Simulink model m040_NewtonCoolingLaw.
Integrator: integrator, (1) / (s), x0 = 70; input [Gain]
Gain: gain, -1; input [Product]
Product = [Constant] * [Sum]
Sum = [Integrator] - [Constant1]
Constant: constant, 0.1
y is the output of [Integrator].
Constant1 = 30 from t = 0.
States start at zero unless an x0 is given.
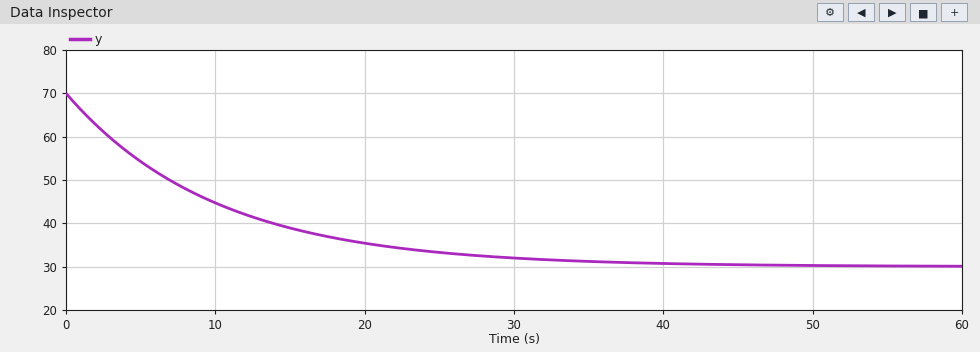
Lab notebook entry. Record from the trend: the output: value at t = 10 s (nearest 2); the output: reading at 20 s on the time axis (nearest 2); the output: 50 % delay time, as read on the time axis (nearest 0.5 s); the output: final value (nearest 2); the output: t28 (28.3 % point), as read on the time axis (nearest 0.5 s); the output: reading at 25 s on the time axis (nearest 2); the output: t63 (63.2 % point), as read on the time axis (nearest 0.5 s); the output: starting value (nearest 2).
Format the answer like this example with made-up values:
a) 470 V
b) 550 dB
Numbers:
a) 44
b) 36
c) 7.0 s
d) 30
e) 3.5 s
f) 34
g) 10.0 s
h) 70
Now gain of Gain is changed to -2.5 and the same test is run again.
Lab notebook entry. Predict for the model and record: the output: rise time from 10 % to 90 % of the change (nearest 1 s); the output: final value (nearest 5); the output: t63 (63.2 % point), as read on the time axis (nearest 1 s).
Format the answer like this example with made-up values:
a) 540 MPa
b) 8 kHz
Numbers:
a) 9 s
b) 30
c) 4 s
